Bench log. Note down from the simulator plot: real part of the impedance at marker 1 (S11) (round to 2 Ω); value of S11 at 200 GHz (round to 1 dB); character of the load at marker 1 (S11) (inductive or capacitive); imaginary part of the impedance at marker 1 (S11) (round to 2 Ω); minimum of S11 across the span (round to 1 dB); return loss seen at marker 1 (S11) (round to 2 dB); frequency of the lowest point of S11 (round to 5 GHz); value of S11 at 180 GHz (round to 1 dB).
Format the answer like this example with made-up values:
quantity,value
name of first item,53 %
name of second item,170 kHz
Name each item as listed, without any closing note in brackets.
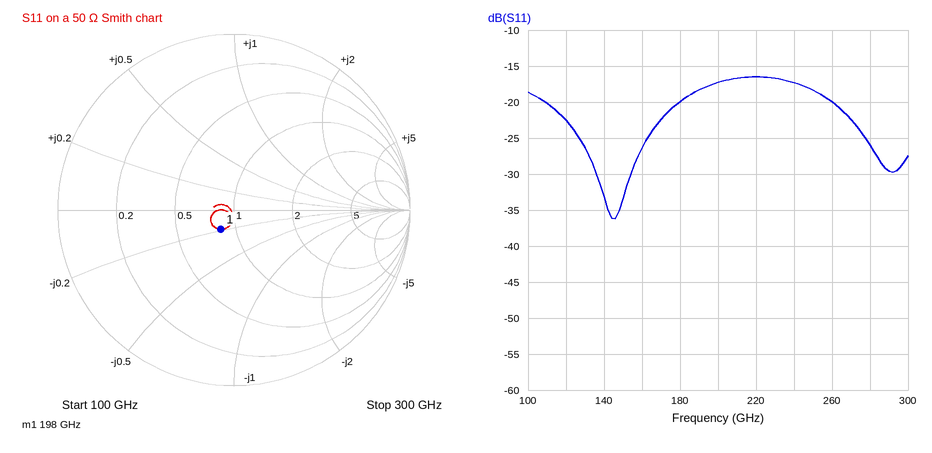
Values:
quantity,value
real part of the impedance at marker 1 (S11),42 Ω
value of S11 at 200 GHz,-17 dB
character of the load at marker 1 (S11),capacitive
imaginary part of the impedance at marker 1 (S11),-10 Ω
minimum of S11 across the span,-36 dB
return loss seen at marker 1 (S11),18 dB
frequency of the lowest point of S11,145 GHz
value of S11 at 180 GHz,-20 dB
